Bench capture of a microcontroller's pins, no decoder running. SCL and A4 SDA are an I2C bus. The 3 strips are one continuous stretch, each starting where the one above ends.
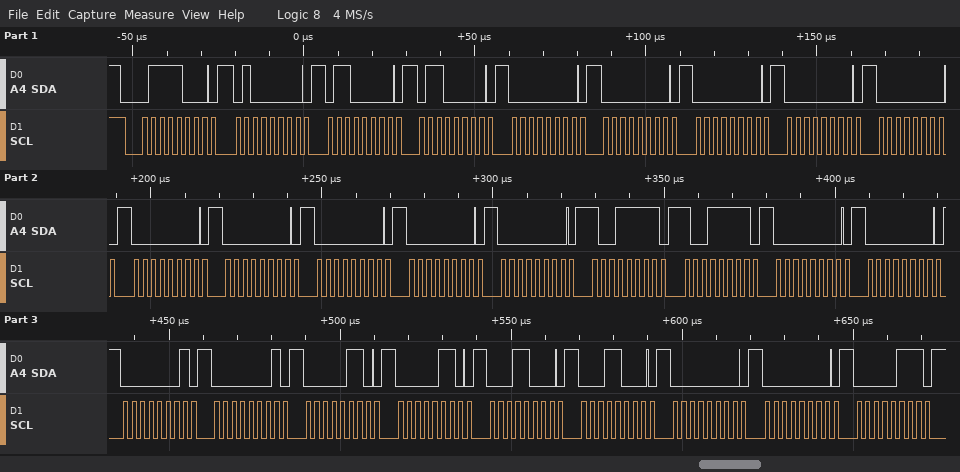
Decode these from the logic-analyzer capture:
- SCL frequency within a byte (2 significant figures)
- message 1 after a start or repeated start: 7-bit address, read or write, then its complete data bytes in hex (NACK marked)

400 kHz
0x3C write: 40 60 60 00 00 00 00 00 00 00 00 00 00 9F 9F 00 00 01 01 06 06 18 18 00 00 07
